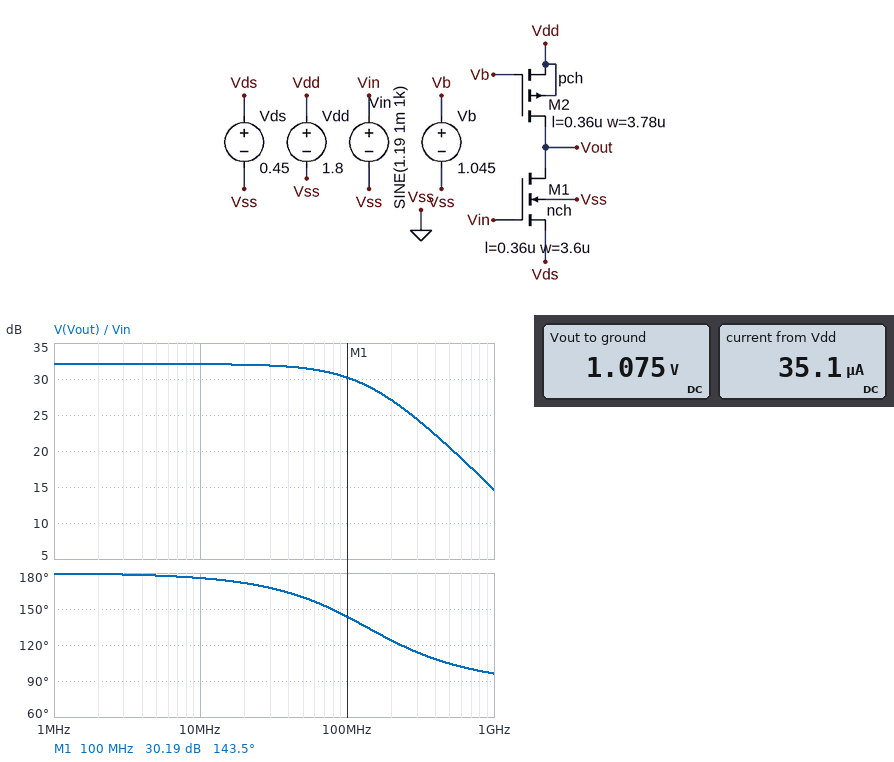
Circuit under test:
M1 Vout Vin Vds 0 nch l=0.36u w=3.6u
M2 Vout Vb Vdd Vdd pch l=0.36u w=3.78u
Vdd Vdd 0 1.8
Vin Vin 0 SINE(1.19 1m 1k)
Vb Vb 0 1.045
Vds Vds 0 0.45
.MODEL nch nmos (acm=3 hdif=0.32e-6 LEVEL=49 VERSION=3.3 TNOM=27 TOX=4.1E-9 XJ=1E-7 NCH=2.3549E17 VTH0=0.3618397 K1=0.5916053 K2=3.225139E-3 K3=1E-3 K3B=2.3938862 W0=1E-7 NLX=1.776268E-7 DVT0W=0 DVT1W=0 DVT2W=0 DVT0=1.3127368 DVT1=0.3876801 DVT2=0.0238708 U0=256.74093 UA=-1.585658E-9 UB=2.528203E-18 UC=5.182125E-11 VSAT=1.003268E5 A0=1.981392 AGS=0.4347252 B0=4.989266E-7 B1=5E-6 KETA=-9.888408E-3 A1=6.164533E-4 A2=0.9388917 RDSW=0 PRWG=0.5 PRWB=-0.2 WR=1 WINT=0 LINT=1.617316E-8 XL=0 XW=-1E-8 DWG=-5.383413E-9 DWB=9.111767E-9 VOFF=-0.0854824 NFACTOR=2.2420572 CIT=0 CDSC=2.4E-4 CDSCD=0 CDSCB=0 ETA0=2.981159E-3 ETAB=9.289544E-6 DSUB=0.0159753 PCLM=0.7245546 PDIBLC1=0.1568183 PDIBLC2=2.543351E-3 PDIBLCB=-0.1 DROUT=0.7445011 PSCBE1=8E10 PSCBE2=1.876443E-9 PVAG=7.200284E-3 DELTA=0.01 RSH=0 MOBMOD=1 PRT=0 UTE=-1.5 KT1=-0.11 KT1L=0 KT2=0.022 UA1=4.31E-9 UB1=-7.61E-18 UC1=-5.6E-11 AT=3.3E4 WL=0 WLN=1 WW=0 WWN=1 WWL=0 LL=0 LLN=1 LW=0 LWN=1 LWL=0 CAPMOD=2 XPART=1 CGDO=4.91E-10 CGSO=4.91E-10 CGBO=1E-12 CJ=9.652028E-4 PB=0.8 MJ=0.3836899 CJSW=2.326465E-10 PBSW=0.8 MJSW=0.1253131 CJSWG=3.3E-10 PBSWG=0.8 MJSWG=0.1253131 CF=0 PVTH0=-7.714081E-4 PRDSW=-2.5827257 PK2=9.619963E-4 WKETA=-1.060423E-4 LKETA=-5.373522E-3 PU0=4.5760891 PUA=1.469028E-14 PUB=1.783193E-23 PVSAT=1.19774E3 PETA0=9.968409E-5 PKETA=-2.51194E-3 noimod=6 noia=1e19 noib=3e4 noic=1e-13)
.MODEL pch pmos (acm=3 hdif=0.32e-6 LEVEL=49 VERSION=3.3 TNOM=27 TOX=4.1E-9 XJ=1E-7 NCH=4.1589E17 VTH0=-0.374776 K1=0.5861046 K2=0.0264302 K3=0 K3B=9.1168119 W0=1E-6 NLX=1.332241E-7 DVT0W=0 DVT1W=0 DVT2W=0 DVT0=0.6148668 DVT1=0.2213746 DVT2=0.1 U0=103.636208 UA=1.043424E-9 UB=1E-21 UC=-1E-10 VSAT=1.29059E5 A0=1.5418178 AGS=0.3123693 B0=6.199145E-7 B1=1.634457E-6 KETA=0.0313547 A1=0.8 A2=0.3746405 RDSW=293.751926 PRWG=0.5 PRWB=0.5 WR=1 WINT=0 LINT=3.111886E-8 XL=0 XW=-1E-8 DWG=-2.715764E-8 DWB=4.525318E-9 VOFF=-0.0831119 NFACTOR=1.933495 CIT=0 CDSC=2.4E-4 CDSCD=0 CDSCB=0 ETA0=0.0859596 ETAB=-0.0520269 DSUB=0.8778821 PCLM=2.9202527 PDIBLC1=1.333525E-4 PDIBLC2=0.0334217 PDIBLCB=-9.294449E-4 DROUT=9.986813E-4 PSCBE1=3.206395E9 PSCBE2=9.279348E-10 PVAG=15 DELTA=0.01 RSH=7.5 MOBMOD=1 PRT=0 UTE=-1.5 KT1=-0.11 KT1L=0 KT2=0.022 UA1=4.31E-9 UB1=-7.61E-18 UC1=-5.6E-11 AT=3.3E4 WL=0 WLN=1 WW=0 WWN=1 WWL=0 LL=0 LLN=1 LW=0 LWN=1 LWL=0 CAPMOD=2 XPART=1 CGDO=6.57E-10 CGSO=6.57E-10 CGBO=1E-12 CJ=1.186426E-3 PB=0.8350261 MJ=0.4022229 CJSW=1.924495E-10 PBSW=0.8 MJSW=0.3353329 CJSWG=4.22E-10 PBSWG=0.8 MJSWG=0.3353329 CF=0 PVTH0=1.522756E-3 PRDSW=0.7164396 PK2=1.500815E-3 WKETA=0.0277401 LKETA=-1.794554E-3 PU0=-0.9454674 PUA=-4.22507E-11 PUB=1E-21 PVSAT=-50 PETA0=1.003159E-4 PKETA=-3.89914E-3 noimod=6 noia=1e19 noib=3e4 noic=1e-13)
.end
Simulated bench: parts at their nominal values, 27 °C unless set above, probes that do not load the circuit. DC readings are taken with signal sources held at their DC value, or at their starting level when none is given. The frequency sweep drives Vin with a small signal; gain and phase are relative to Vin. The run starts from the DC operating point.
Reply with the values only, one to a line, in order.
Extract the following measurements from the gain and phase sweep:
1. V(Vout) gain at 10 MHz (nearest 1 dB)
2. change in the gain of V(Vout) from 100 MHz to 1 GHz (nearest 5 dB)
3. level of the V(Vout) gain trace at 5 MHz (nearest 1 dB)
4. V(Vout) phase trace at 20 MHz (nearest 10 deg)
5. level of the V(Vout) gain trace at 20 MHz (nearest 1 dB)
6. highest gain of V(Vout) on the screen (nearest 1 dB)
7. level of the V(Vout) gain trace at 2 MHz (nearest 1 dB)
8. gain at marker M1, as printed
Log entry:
32 dB
-15 dB
32 dB
170 deg
32 dB
32 dB
32 dB
30.19 dB
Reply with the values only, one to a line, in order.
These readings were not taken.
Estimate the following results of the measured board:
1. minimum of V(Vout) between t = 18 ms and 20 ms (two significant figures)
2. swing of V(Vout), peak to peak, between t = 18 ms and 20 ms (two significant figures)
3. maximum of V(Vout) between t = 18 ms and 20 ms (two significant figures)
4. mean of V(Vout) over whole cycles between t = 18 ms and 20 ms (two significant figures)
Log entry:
1.0 V
80 mV
1.1 V
1.1 V
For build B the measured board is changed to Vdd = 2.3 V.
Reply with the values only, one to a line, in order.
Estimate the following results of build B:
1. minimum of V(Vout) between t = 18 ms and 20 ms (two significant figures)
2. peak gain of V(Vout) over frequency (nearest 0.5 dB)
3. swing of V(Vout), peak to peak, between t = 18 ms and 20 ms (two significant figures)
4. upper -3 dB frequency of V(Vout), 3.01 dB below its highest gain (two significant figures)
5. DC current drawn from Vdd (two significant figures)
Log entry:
2.2 V
-1.0 dB
1.8 mV
3.2 GHz
41 µA
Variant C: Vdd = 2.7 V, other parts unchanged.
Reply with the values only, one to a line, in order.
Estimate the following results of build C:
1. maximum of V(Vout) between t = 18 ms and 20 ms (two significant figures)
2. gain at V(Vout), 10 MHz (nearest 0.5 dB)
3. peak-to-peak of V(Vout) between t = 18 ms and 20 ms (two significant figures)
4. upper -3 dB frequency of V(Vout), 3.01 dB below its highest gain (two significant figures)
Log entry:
2.6 V
-4.0 dB
1.3 mV
4.6 GHz
